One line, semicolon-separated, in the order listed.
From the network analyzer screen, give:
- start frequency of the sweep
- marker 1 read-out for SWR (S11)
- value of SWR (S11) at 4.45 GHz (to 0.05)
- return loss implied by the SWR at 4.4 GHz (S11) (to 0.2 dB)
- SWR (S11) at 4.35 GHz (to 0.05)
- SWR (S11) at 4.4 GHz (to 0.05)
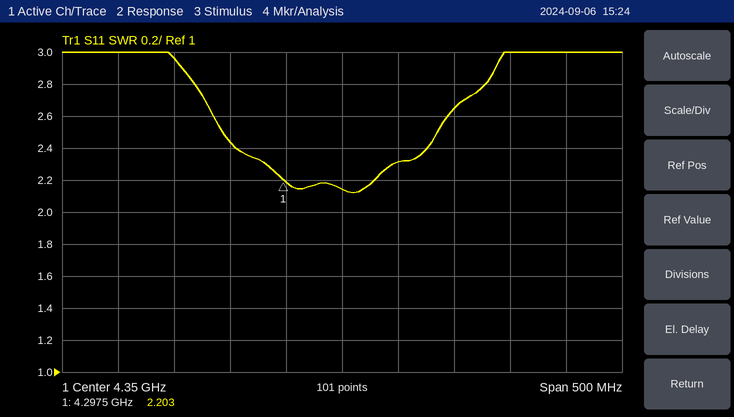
4.1 GHz; 2.203; 2.65; 8.0 dB; 2.15; 2.30
